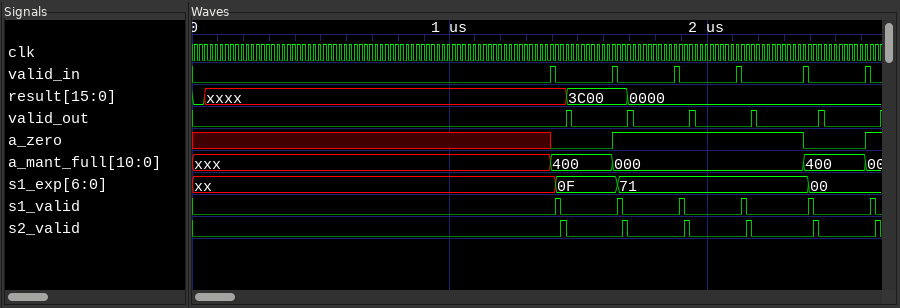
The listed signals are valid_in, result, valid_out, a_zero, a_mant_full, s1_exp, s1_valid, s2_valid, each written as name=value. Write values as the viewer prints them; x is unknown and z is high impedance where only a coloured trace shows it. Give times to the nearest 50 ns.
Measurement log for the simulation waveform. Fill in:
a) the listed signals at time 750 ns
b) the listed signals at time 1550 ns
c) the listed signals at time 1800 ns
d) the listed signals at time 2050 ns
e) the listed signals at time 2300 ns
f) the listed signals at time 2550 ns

valid_in=0, result=xxxx, valid_out=0, a_zero=x, a_mant_full=xxx, s1_exp=xx, s1_valid=0, s2_valid=0
valid_in=0, result=3C00, valid_out=0, a_zero=0, a_mant_full=400, s1_exp=0F, s1_valid=0, s2_valid=0
valid_in=0, result=0000, valid_out=0, a_zero=1, a_mant_full=000, s1_exp=71, s1_valid=0, s2_valid=0
valid_in=0, result=0000, valid_out=0, a_zero=1, a_mant_full=000, s1_exp=71, s1_valid=0, s2_valid=0
valid_in=0, result=0000, valid_out=0, a_zero=1, a_mant_full=000, s1_exp=71, s1_valid=0, s2_valid=0
valid_in=0, result=0000, valid_out=0, a_zero=0, a_mant_full=400, s1_exp=00, s1_valid=0, s2_valid=0
